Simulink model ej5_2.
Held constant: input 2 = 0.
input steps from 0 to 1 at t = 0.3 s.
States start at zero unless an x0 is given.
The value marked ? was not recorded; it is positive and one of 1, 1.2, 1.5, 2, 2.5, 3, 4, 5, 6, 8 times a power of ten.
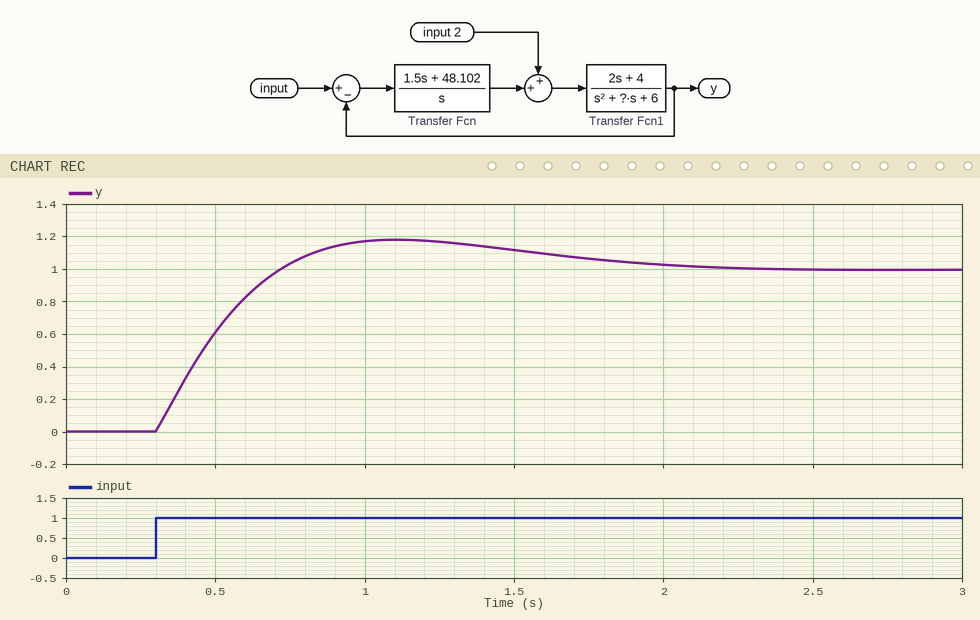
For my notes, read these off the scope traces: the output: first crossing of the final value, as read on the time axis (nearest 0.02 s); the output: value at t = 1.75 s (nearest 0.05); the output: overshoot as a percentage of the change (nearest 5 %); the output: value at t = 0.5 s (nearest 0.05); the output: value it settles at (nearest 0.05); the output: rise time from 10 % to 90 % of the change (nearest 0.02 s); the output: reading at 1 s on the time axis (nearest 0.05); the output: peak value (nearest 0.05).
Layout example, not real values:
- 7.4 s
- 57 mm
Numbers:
- 0.72 s
- 1.05
- 20 %
- 0.60
- 1.00
- 0.32 s
- 1.15
- 1.20
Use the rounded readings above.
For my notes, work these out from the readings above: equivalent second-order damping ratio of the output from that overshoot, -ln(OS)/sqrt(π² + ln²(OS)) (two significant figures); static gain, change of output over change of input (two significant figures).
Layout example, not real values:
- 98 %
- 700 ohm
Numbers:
- 0.46
- 1.0
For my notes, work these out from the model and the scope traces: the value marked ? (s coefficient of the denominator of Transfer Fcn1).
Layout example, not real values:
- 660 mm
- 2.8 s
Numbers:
- 25
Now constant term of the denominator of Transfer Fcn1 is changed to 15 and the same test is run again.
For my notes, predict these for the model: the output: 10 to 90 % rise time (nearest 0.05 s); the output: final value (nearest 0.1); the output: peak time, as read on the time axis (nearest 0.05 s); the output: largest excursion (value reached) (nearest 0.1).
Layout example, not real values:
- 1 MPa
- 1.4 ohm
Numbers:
- 0.35 s
- 1.0
- 1.15 s
- 1.1
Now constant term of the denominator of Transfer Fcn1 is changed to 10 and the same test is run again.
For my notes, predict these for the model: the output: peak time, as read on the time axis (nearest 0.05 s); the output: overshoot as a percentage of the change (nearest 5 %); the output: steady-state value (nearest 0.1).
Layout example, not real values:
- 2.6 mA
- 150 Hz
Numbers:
- 1.10 s
- 15 %
- 1.0
